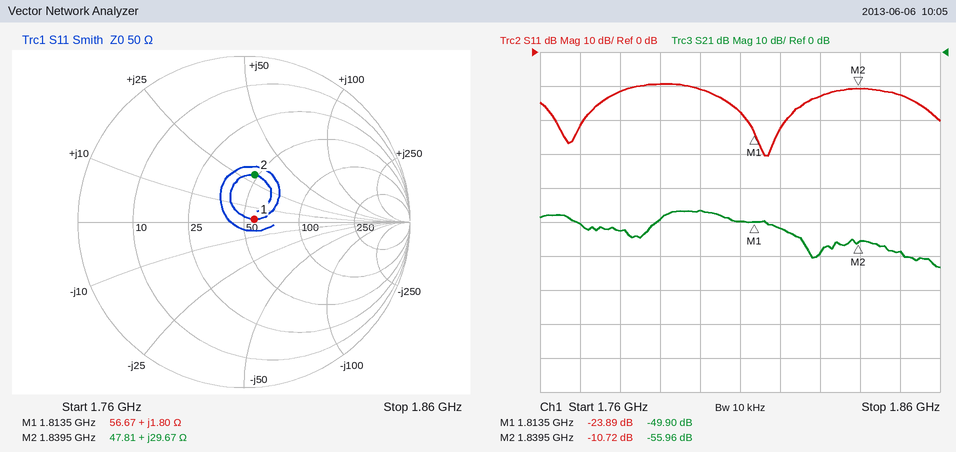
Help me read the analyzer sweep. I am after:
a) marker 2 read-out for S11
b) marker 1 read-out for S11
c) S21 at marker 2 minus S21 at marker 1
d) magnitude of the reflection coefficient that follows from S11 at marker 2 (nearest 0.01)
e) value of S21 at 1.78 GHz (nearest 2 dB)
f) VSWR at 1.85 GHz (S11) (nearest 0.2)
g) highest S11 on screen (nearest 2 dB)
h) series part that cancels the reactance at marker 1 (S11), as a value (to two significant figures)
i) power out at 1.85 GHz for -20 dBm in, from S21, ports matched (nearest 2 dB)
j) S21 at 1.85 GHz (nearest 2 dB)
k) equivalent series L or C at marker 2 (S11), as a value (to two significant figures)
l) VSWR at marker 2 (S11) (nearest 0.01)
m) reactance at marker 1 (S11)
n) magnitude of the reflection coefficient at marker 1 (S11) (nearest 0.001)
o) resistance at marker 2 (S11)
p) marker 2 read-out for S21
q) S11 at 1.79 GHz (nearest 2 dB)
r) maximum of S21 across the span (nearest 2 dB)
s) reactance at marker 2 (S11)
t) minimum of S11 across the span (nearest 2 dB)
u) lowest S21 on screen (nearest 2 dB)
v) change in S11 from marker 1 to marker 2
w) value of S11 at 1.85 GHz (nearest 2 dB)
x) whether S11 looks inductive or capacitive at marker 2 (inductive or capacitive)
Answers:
-10.72 dB
-23.89 dB
-6.06 dB
0.29
-52 dB
1.6
-10 dB
49 pF
-78 dBm
-58 dB
2.6 nH
1.82
+1.80 Ω
0.064
47.81 Ω
-55.96 dB
-10 dB
-46 dB
+29.67 Ω
-30 dB
-64 dB
13.17 dB
-12 dB
inductive
